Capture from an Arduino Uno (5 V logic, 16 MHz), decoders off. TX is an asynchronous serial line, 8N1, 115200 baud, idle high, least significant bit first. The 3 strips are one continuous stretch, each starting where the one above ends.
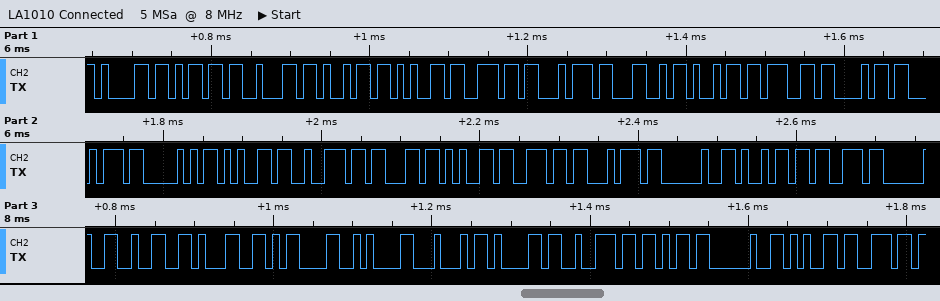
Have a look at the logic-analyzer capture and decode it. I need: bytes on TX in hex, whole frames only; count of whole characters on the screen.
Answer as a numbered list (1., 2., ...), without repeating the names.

1. 61 6D 62 69 65 6E 74 4C 69 67 68 74 50 65 72 63 65 6E 74 20 69 73 20 32 31 0D 0A 44 61 72 6B 20 65 6E
2. 34
